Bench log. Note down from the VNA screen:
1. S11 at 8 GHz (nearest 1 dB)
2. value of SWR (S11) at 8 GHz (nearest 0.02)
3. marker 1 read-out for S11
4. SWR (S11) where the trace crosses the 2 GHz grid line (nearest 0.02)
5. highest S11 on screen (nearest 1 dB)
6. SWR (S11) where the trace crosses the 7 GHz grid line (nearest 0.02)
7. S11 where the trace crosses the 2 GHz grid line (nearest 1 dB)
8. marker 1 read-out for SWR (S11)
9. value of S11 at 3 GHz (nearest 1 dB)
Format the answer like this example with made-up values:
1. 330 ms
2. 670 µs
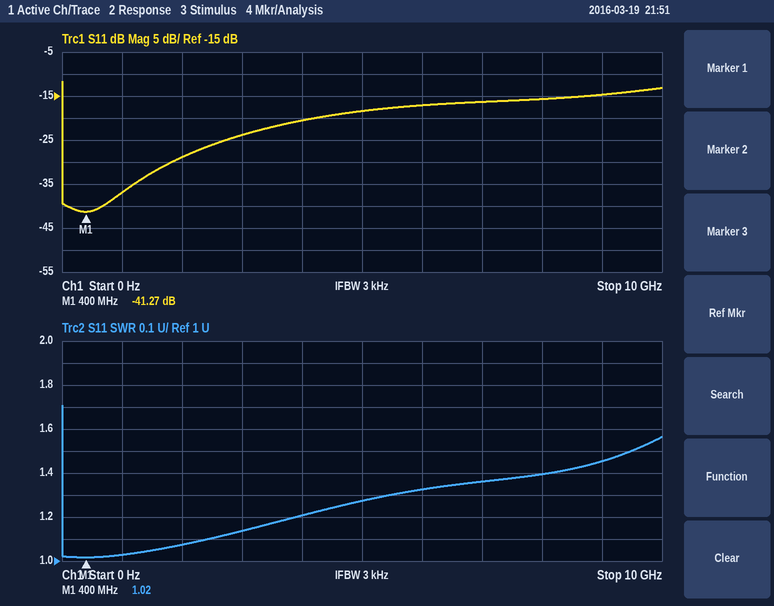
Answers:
1. -16 dB
2. 1.40
3. -41.27 dB
4. 1.08
5. -12 dB
6. 1.36
7. -29 dB
8. 1.02
9. -24 dB
